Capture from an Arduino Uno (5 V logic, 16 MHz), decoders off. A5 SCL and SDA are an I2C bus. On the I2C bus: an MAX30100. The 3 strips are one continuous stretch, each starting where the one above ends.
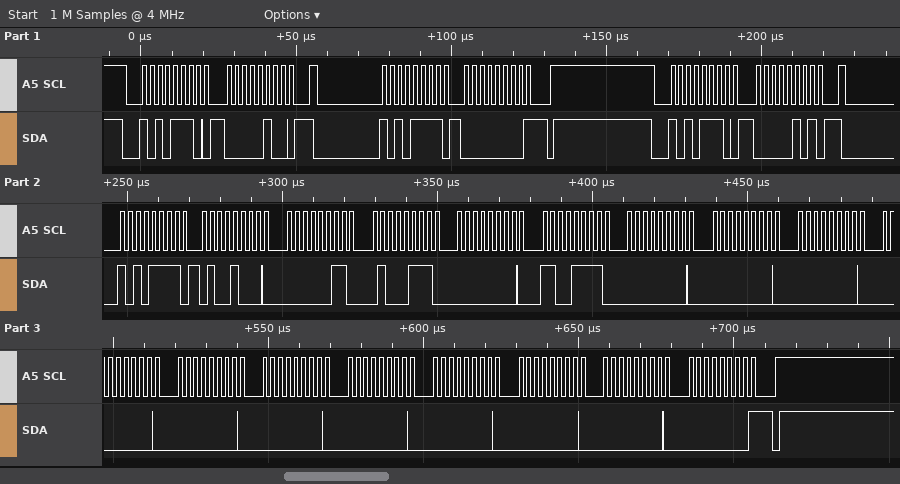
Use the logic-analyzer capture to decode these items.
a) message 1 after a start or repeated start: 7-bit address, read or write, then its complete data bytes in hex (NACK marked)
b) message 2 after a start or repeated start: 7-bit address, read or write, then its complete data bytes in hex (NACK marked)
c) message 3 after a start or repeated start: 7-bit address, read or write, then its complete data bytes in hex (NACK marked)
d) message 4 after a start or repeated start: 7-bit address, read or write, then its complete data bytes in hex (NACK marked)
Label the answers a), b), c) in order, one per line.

a) 0x57 write: 04
b) 0x57 read: 00 NACK
c) 0x57 write: 05
d) 0x57 read: 48 03 47 00 CF 00 00 00 00 00 00 00 00 00 00 00 NACK
